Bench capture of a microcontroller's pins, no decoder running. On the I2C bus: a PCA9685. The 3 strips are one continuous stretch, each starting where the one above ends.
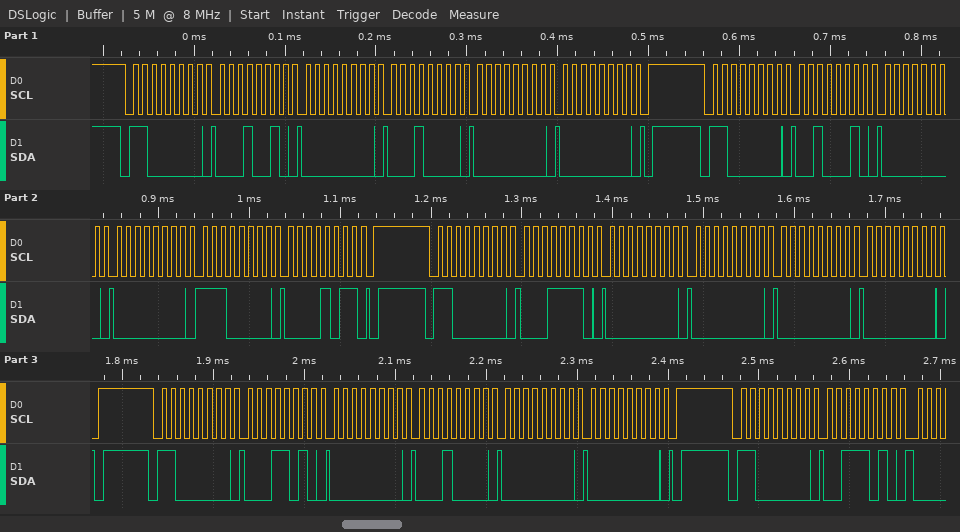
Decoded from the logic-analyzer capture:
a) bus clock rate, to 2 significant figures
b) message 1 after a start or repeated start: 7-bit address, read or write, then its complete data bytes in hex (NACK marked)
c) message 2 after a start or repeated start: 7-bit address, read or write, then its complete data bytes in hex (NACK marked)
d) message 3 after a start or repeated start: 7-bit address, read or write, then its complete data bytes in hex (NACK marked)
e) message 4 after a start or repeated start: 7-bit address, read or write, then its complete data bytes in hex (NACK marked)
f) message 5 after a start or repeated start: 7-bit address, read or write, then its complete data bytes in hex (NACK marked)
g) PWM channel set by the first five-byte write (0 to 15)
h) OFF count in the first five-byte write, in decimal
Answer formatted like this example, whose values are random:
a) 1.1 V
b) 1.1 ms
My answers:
a) 100 kHz
b) 0x60 write: 12 00 10 00 00
c) 0x60 write: 22 00 00 E0 0B
d) 0x60 write: 1E 00 00 00 00
e) 0x60 write: 1A 00 10 00 00
f) 0x60 write: 3A
g) 3
h) 0
